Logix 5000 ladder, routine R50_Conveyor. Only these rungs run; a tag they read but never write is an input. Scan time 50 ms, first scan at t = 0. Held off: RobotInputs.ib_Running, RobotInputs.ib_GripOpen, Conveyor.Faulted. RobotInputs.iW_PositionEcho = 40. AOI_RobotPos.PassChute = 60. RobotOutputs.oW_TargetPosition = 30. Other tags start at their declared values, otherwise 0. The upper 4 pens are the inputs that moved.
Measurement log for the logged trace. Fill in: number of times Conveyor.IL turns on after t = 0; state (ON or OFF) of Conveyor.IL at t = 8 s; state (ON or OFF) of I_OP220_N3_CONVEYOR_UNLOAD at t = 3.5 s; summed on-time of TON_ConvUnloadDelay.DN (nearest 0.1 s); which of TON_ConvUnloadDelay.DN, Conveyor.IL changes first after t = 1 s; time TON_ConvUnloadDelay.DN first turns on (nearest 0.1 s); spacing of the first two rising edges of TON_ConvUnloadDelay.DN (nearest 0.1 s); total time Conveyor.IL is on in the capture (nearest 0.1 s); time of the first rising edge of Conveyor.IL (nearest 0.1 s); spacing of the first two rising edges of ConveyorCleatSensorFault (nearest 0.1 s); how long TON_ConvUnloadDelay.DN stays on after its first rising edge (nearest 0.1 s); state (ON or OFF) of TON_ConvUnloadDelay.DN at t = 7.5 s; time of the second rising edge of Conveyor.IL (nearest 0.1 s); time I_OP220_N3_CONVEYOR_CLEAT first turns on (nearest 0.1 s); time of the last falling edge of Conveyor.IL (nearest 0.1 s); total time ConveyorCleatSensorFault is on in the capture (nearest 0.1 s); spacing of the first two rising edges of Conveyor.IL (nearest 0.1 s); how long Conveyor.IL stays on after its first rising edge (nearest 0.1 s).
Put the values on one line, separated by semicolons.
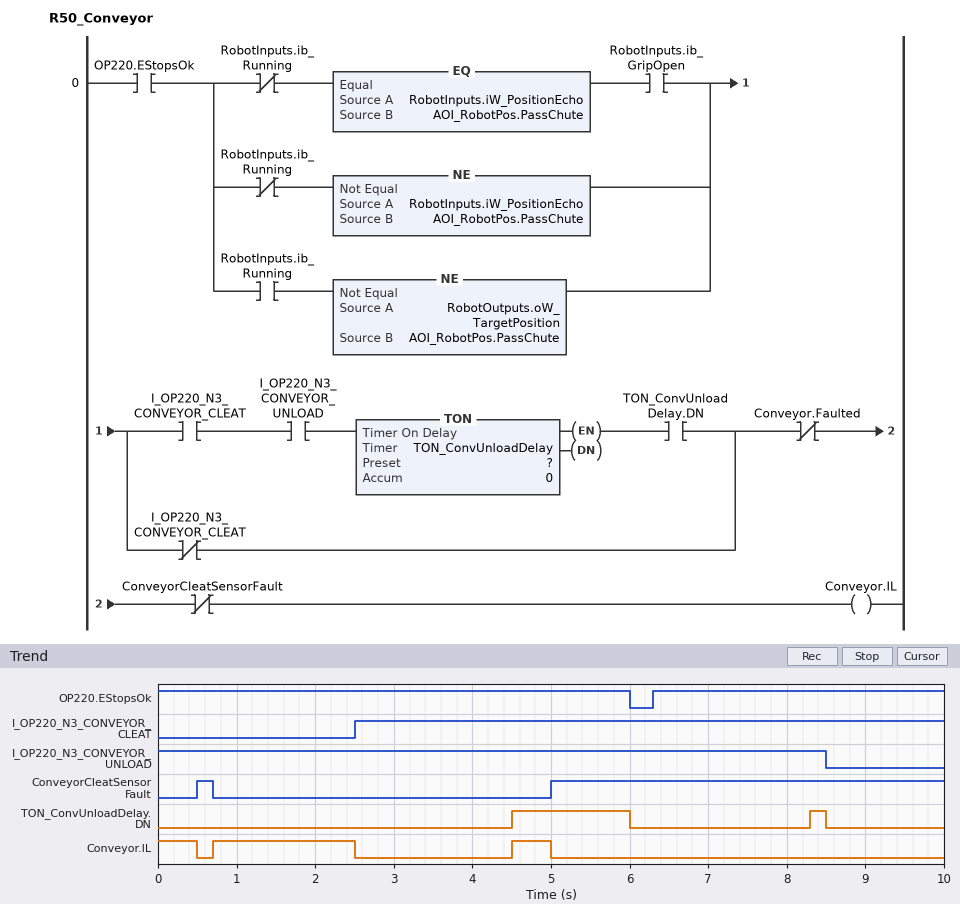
2; OFF; ON; 1.7 s; Conveyor.IL; 4.5 s; 3.8 s; 2.8 s; 0.7 s; 4.5 s; 1.5 s; OFF; 4.5 s; 2.5 s; 5.0 s; 5.2 s; 3.8 s; 1.8 s
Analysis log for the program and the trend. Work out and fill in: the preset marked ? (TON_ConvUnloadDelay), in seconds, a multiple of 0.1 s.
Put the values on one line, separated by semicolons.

2.0 s
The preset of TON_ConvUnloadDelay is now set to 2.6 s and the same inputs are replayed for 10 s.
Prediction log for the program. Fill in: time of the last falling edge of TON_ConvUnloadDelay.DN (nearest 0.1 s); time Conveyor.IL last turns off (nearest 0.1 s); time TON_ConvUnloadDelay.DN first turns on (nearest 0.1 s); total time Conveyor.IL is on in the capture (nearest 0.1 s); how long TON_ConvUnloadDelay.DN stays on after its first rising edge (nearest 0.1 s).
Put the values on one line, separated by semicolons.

6.0 s; 2.5 s; 5.1 s; 2.3 s; 0.9 s
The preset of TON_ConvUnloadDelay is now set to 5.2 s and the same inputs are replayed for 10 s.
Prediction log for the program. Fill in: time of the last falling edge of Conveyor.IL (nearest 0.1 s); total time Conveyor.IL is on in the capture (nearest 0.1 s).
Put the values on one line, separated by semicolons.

2.5 s; 2.3 s
